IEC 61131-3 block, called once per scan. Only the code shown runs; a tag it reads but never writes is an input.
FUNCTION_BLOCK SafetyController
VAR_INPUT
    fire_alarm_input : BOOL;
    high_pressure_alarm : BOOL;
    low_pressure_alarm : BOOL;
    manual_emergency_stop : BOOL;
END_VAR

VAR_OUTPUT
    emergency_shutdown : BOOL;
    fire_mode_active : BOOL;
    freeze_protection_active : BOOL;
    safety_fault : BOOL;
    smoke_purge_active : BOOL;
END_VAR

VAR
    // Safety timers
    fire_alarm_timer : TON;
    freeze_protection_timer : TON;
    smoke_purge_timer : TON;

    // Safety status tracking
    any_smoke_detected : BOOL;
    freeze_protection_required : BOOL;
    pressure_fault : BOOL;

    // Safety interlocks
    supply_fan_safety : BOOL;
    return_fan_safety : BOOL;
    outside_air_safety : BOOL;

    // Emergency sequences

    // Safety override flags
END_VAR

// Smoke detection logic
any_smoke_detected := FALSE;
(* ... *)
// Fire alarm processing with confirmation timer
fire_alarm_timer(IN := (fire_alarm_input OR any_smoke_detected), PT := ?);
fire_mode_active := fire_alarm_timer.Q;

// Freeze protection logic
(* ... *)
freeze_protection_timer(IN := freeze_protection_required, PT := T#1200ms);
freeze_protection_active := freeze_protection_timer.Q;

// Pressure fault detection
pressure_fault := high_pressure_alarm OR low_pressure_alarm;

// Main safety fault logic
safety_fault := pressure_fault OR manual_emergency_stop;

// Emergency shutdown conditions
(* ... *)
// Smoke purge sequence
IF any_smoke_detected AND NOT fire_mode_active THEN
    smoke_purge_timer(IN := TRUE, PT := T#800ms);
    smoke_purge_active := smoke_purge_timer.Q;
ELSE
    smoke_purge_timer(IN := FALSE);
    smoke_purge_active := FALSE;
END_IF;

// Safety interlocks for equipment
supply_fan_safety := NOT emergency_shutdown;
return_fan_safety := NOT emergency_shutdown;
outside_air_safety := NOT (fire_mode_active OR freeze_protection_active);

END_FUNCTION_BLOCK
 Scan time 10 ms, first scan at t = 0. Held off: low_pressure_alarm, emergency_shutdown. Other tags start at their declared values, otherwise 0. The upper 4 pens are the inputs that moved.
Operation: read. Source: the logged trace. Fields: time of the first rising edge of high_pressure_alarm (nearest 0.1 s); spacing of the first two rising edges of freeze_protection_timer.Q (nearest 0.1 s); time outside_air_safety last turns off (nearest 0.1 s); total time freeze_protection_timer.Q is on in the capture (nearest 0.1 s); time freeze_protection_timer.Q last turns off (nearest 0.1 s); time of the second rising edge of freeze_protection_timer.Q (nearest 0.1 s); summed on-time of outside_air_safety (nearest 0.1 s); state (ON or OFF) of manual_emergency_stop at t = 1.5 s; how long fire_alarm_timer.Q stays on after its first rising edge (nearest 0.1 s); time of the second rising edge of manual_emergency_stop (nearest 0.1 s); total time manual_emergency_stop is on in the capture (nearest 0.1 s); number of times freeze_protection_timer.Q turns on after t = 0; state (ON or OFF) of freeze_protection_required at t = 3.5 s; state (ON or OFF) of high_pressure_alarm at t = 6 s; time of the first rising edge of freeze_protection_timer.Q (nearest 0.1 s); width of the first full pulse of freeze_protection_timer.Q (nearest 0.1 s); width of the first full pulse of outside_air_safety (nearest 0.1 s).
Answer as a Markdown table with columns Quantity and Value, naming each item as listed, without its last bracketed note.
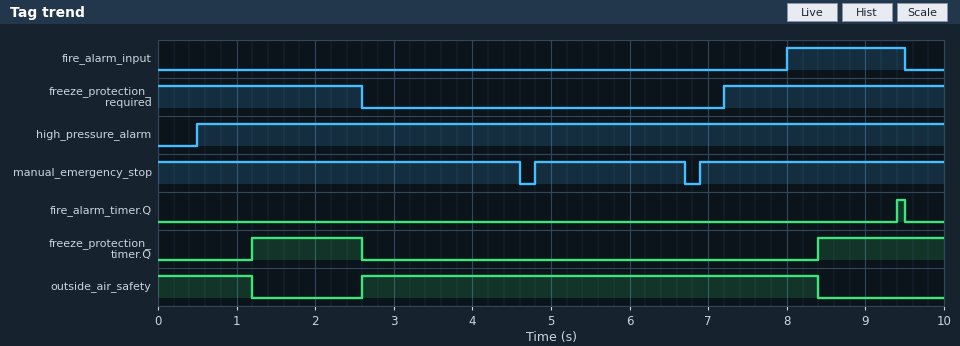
| Quantity | Value |
|---|---|
| time of the first rising edge of high_pressure_alarm | 0.5 s |
| spacing of the first two rising edges of freeze_protection_timer.Q | 7.2 s |
| time outside_air_safety last turns off | 8.4 s |
| total time freeze_protection_timer.Q is on in the capture | 3.0 s |
| time freeze_protection_timer.Q last turns off | 2.6 s |
| time of the second rising edge of freeze_protection_timer.Q | 8.4 s |
| summed on-time of outside_air_safety | 7.0 s |
| state (ON or OFF) of manual_emergency_stop at t = 1.5 s | ON |
| how long fire_alarm_timer.Q stays on after its first rising edge | 0.1 s |
| time of the second rising edge of manual_emergency_stop | 6.9 s |
| total time manual_emergency_stop is on in the capture | 9.6 s |
| number of times freeze_protection_timer.Q turns on after t = 0 | 2 |
| state (ON or OFF) of freeze_protection_required at t = 3.5 s | OFF |
| state (ON or OFF) of high_pressure_alarm at t = 6 s | ON |
| time of the first rising edge of freeze_protection_timer.Q | 1.2 s |
| width of the first full pulse of freeze_protection_timer.Q | 1.4 s |
| width of the first full pulse of outside_air_safety | 5.8 s |
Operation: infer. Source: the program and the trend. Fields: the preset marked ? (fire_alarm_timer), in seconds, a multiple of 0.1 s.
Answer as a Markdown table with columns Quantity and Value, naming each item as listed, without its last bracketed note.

| Quantity | Value |
|---|---|
| the preset marked ? (fire_alarm_timer), in seconds, a multiple of 0.1 s | 1.4 s |
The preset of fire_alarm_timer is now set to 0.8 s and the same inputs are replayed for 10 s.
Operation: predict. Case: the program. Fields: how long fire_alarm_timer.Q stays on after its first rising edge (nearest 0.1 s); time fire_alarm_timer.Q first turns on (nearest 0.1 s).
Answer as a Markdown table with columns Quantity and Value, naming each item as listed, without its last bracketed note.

| Quantity | Value |
|---|---|
| how long fire_alarm_timer.Q stays on after its first rising edge | 0.7 s |
| time fire_alarm_timer.Q first turns on | 8.8 s |
